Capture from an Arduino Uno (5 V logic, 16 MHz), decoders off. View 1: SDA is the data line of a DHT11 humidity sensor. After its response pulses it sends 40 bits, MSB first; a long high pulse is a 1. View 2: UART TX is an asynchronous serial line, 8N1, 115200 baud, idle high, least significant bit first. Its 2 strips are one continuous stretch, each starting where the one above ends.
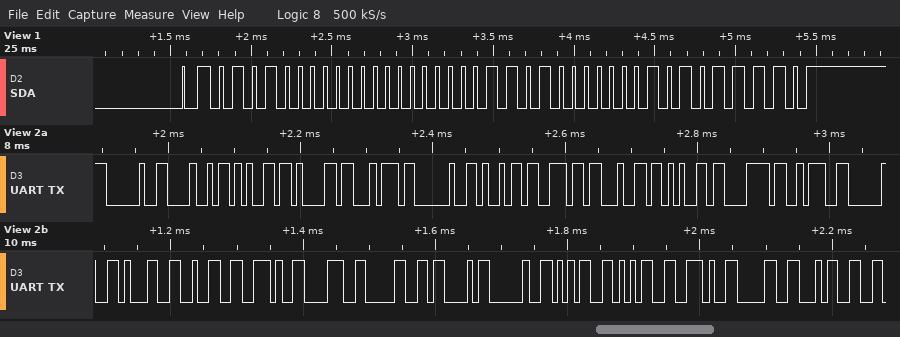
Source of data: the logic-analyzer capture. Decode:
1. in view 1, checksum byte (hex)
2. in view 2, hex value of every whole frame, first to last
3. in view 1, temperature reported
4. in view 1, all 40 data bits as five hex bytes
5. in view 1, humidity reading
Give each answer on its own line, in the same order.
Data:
0x5E
20 48 65 61 74 20 69 6E 64 65 78 3A 20 31 32 2E 38 30 43 20 35 35 2E 30 34
13.1 °C
50 00 0D 01 5E
80 %
